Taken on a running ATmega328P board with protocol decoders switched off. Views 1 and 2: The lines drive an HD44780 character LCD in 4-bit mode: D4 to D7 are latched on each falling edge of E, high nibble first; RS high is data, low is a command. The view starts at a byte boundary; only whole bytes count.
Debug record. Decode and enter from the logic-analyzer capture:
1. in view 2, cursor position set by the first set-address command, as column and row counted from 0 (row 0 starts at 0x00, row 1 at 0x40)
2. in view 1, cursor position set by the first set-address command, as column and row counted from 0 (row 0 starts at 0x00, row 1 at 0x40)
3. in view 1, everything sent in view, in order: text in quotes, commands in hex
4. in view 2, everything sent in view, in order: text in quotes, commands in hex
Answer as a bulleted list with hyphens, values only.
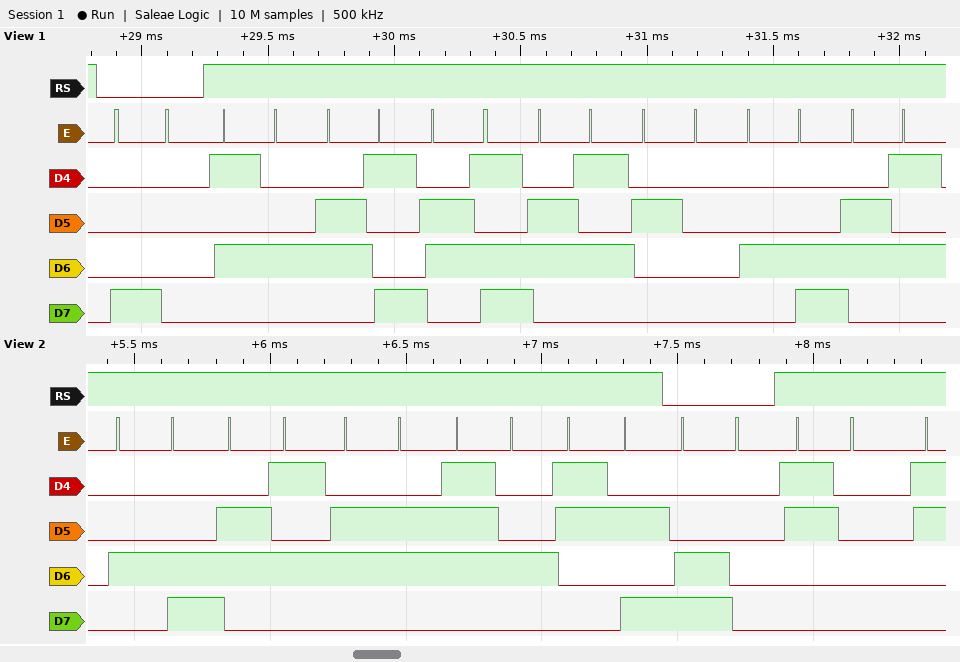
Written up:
- column 0, row 1
- column 0, row 0
- 0x80 "Time Le"
- "Left:" 0xC0 "0"
